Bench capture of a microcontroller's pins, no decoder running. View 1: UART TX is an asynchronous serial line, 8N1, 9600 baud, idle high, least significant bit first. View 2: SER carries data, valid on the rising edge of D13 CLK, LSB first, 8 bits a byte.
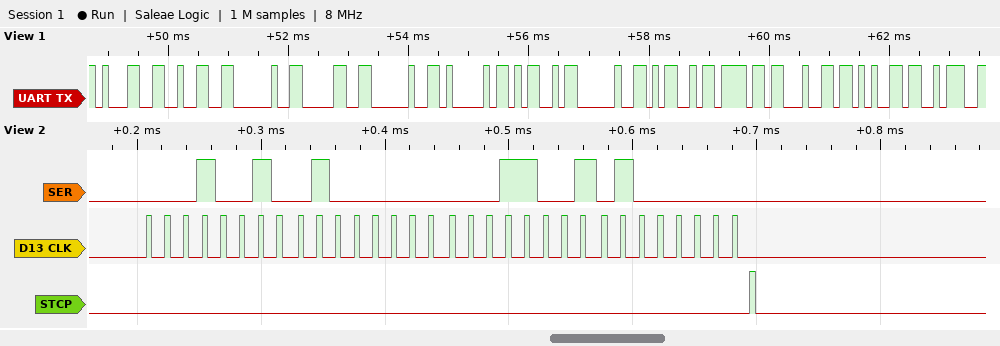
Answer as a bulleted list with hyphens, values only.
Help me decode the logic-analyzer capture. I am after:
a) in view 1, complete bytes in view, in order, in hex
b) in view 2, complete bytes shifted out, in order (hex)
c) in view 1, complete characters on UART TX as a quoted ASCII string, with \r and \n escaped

- 0x31 0x32 0x20 0x30 0x20 0x41 0x4D 0x20 0x4D 0x6F 0x64 0x65 0x3A
- 48 02 98 02
- "12 0 AM Mode:"
